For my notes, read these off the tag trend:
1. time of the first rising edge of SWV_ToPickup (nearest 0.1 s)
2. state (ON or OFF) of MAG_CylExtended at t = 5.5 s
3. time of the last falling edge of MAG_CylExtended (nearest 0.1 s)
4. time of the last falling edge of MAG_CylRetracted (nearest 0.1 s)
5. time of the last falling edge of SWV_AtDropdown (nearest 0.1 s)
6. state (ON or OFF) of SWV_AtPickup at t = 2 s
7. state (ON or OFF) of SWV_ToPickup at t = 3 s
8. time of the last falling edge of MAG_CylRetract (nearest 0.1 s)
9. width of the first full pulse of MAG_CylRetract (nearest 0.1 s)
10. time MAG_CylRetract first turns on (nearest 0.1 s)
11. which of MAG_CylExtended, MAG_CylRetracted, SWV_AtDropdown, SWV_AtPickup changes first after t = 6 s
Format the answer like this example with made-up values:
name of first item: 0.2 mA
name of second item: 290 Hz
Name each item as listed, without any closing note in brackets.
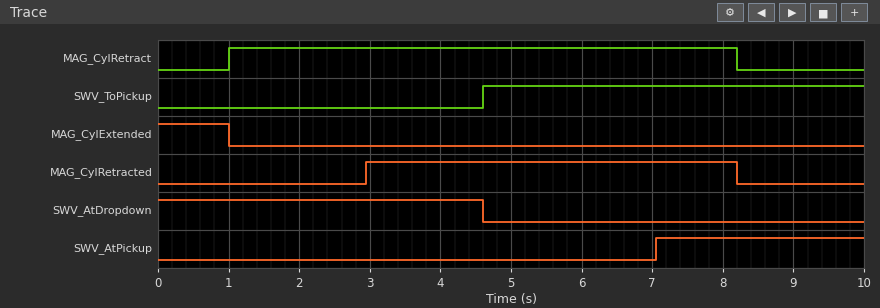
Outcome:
time of the first rising edge of SWV_ToPickup: 4.6 s
state (ON or OFF) of MAG_CylExtended at t = 5.5 s: OFF
time of the last falling edge of MAG_CylExtended: 1.0 s
time of the last falling edge of MAG_CylRetracted: 8.2 s
time of the last falling edge of SWV_AtDropdown: 4.6 s
state (ON or OFF) of SWV_AtPickup at t = 2 s: OFF
state (ON or OFF) of SWV_ToPickup at t = 3 s: OFF
time of the last falling edge of MAG_CylRetract: 8.2 s
width of the first full pulse of MAG_CylRetract: 7.2 s
time MAG_CylRetract first turns on: 1.0 s
which of MAG_CylExtended, MAG_CylRetracted, SWV_AtDropdown, SWV_AtPickup changes first after t = 6 s: SWV_AtPickup
